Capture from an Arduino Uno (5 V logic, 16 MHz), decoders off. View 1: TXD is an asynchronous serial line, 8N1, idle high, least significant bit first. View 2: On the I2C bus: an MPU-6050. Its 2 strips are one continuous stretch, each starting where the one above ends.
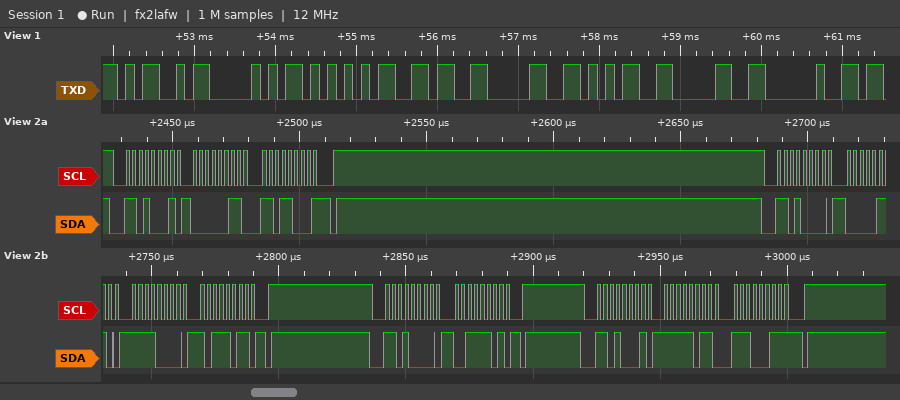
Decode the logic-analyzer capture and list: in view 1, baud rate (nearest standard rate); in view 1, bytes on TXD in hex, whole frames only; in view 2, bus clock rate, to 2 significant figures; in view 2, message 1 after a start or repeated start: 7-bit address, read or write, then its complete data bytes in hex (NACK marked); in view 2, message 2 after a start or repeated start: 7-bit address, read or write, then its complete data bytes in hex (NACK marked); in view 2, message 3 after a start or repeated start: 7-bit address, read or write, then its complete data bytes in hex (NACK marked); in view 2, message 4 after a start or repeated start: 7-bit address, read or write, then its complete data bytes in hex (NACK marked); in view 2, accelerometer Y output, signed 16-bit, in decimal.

9600 baud
0x4D 0x50 0x55 0x36 0x30 0x35 0x30 0x20
400 kHz
0x68 read: 03 D8 NACK
0x68 write: 06 F0 BB
0x68 write: 3D
0x68 read: FB E3 NACK
-1053
